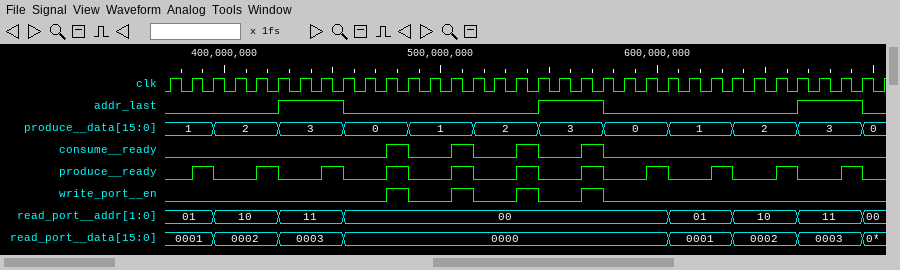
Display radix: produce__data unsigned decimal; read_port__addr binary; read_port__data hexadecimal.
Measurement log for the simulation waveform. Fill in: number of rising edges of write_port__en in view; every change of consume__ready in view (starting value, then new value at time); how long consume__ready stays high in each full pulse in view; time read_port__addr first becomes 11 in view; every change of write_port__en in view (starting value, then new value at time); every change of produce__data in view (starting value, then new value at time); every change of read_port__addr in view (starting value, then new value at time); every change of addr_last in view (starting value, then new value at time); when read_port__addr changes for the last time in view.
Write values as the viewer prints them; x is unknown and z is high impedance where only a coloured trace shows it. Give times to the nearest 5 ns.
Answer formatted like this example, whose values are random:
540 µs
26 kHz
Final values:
4
0, 1 at 475 ns, 0 at 485 ns, 1 at 505 ns, 0 at 515 ns, 1 at 535 ns, 0 at 545 ns, 1 at 565 ns, 0 at 575 ns
10 ns, 10 ns, 10 ns, 10 ns
425 ns
0, 1 at 475 ns, 0 at 485 ns, 1 at 505 ns, 0 at 515 ns, 1 at 535 ns, 0 at 545 ns, 1 at 565 ns, 0 at 575 ns
1, 2 at 395 ns, 3 at 425 ns, 0 at 455 ns, 1 at 485 ns, 2 at 515 ns, 3 at 545 ns, 0 at 575 ns, 1 at 605 ns, 2 at 635 ns, 3 at 665 ns, 0 at 695 ns
01, 10 at 395 ns, 11 at 425 ns, 00 at 455 ns, 01 at 605 ns, 10 at 635 ns, 11 at 665 ns, 00 at 695 ns
0, 1 at 425 ns, 0 at 455 ns, 1 at 545 ns, 0 at 575 ns, 1 at 665 ns, 0 at 695 ns
695 ns
